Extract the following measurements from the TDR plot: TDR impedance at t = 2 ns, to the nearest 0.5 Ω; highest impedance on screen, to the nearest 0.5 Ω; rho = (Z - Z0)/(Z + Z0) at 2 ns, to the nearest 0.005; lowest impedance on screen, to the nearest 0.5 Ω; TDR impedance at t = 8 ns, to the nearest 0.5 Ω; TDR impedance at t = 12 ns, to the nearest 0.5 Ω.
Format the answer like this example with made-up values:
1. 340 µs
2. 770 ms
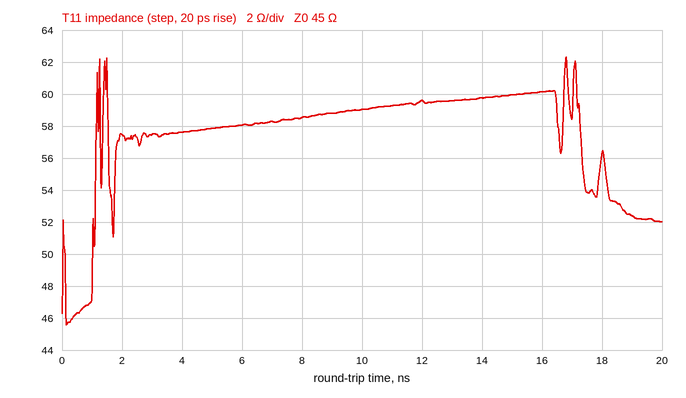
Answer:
1. 57.5 Ω
2. 62.5 Ω
3. +0.120
4. 45.5 Ω
5. 58.5 Ω
6. 59.5 Ω
